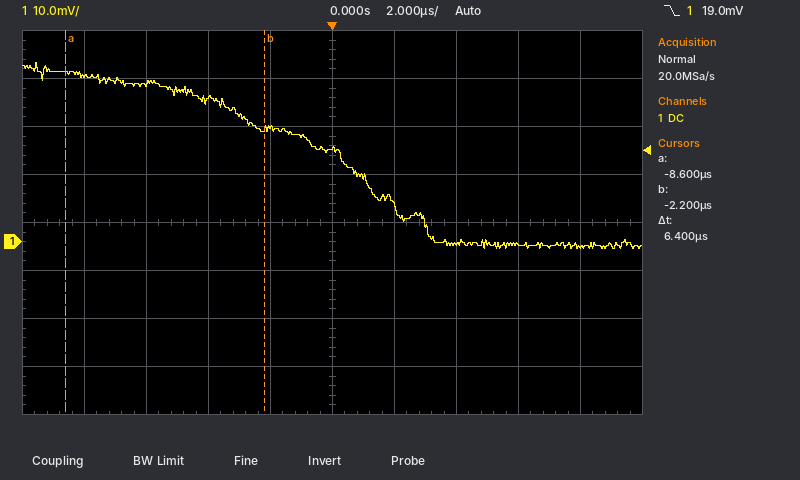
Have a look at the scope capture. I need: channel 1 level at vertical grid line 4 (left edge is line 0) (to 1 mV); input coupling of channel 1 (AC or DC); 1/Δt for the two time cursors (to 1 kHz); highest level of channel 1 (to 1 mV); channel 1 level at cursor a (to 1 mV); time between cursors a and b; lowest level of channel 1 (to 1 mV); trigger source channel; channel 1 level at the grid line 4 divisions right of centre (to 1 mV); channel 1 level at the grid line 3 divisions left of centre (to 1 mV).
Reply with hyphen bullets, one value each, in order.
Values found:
- 24 mV
- DC
- 156 kHz
- 37 mV
- 35 mV
- 6.4 µs
- -1 mV
- channel 1
- -1 mV
- 33 mV
